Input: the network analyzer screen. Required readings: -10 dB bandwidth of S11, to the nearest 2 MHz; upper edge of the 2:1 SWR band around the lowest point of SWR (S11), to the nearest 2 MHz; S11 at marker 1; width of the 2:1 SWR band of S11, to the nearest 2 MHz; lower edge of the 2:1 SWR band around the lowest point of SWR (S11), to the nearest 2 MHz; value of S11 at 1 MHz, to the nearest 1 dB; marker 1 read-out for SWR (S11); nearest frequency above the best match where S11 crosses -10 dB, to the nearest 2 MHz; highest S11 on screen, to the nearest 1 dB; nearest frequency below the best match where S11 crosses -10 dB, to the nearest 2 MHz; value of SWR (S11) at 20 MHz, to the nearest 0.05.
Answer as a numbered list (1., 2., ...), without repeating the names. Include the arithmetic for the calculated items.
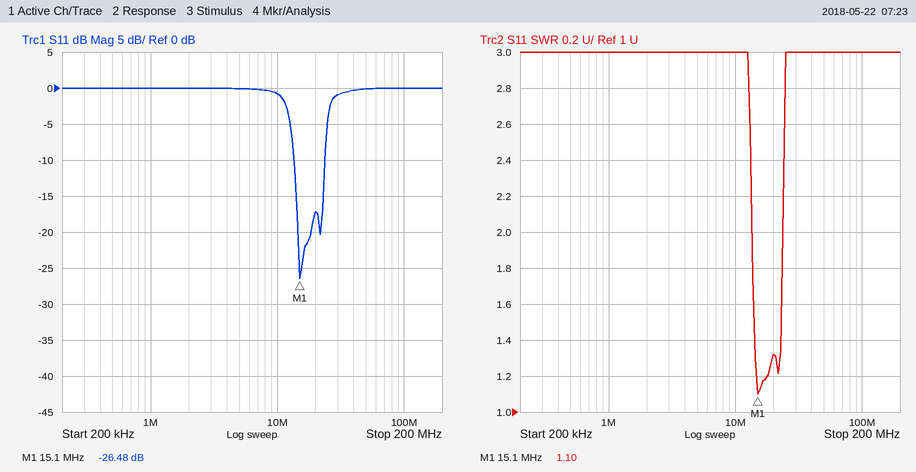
1. 24 MHz − 14 MHz = 10 MHz
2. 24 MHz
3. -26.48 dB
4. 24 MHz − 14 MHz = 10 MHz
5. 14 MHz
6. 0 dB
7. 1.10
8. 24 MHz
9. 0 dB
10. 14 MHz
11. 1.30
